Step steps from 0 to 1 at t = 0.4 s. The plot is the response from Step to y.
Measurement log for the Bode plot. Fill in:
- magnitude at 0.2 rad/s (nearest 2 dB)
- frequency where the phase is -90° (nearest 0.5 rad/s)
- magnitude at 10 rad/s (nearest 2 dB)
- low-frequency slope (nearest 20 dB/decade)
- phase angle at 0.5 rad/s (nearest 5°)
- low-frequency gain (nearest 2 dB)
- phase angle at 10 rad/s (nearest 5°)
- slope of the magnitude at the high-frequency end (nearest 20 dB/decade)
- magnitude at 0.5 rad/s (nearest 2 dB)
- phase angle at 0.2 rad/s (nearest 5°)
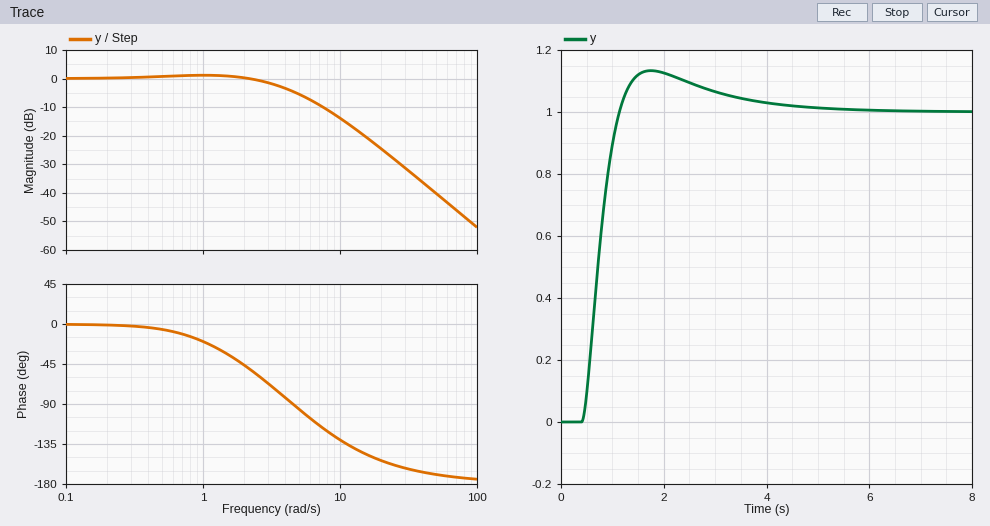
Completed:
0 dB
4.5 rad/s
-14 dB
0 dB/decade
-5°
0 dB
-130°
-40 dB/decade
0 dB
0°
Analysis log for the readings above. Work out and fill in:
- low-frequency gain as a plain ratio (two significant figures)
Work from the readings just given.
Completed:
1.0
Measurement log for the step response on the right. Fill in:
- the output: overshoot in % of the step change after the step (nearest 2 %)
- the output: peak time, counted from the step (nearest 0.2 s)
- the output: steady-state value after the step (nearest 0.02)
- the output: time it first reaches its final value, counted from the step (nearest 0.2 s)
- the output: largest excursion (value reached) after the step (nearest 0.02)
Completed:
14 %
1.4 s
1.00
0.8 s
1.14
